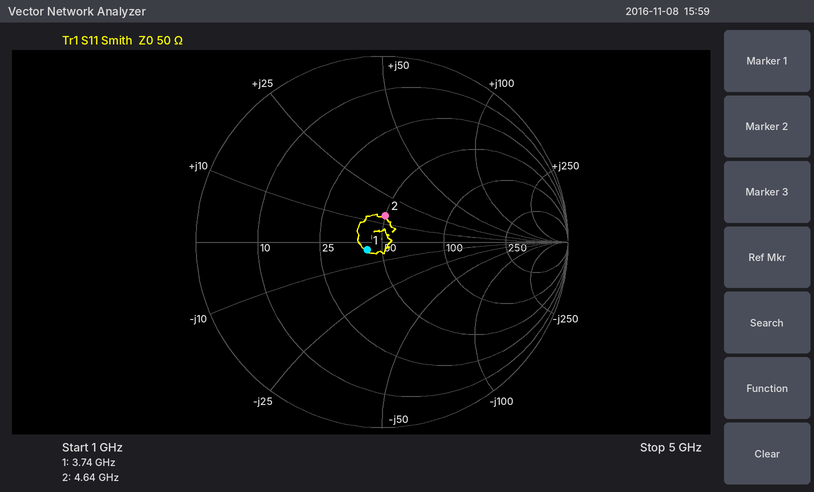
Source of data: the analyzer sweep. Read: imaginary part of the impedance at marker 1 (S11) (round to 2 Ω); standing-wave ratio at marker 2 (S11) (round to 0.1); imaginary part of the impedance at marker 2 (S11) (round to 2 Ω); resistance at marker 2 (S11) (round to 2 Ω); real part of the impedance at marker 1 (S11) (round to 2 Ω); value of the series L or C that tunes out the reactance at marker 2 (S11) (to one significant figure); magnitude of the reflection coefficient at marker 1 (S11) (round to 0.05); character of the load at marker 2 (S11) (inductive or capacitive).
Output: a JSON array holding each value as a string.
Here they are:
["-4 Ω", "1.3", "+14 Ω", "50 Ω", "42 Ω", "2 pF", "0.10", "inductive"]
